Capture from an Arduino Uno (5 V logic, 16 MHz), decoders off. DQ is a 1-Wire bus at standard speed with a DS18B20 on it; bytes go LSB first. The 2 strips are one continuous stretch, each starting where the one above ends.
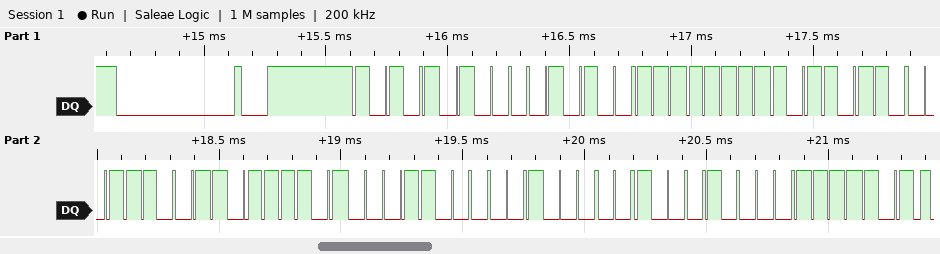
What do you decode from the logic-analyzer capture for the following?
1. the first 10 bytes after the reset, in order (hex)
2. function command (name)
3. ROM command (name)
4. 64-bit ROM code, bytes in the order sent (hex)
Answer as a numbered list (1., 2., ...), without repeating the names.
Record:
1. 55 28 FF 6D 9C BD 18 04 11 BE
2. Read Scratchpad
3. Match ROM
4. 28 FF 6D 9C BD 18 04 11
